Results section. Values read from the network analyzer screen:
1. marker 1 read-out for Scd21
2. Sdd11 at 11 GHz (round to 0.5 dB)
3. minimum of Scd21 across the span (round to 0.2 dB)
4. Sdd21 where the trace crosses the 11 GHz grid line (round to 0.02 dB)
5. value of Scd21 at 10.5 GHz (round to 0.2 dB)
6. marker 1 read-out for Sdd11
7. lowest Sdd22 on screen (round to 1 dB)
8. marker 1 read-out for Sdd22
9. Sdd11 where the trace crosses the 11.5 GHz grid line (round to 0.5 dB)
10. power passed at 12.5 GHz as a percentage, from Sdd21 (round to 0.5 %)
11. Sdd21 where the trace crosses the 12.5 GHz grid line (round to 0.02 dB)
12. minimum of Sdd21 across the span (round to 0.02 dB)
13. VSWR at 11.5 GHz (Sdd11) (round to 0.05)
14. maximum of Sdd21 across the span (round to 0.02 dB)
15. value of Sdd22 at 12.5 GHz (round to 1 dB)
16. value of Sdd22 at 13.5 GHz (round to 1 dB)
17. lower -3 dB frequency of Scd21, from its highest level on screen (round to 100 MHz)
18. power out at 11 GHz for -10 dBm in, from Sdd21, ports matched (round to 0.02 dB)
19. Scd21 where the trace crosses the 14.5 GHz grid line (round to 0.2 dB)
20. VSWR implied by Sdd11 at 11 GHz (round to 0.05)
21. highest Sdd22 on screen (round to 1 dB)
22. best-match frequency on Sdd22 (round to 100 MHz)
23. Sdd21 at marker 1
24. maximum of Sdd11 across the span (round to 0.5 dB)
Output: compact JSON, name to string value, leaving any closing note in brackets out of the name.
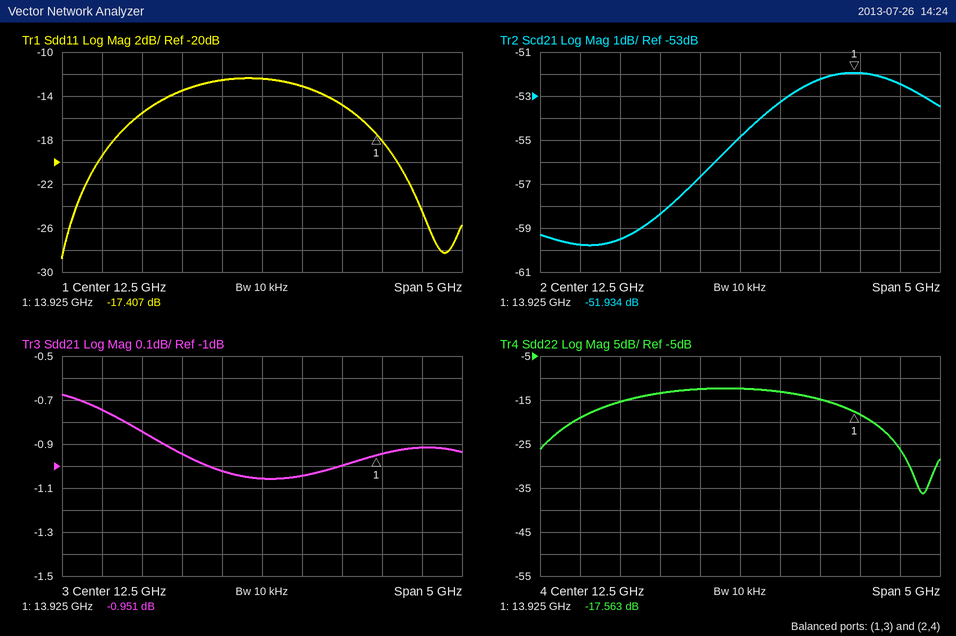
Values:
{"marker 1 read-out for Scd21": "-51.934 dB", "Sdd11 at 11 GHz": "-15.5 dB", "minimum of Scd21 across the span": "-59.8 dB", "Sdd21 where the trace crosses the 11 GHz grid line": "-0.84 dB", "value of Scd21 at 10.5 GHz": "-59.8 dB", "marker 1 read-out for Sdd11": "-17.407 dB", "lowest Sdd22 on screen": "-36 dB", "marker 1 read-out for Sdd22": "-17.563 dB", "Sdd11 where the trace crosses the 11.5 GHz grid line": "-13.5 dB", "power passed at 12.5 GHz as a percentage, from Sdd21": "78.5 %", "Sdd21 where the trace crosses the 12.5 GHz grid line": "-1.06 dB", "minimum of Sdd21 across the span": "-1.06 dB", "VSWR at 11.5 GHz (Sdd11)": "1.55", "maximum of Sdd21 across the span": "-0.68 dB", "value of Sdd22 at 12.5 GHz": "-12 dB", "value of Sdd22 at 13.5 GHz": "-15 dB", "lower -3 dB frequency of Scd21, from its highest level on screen": "12.5 GHz", "power out at 11 GHz for -10 dBm in, from Sdd21, ports matched": "-10.84 dBm", "Scd21 where the trace crosses the 14.5 GHz grid line": "-52.4 dB", "VSWR implied by Sdd11 at 11 GHz": "1.40", "highest Sdd22 on screen": "-12 dB", "best-match frequency on Sdd22": "14.8 GHz", "Sdd21 at marker 1": "-0.951 dB", "maximum of Sdd11 across the span": "-12.5 dB"}
